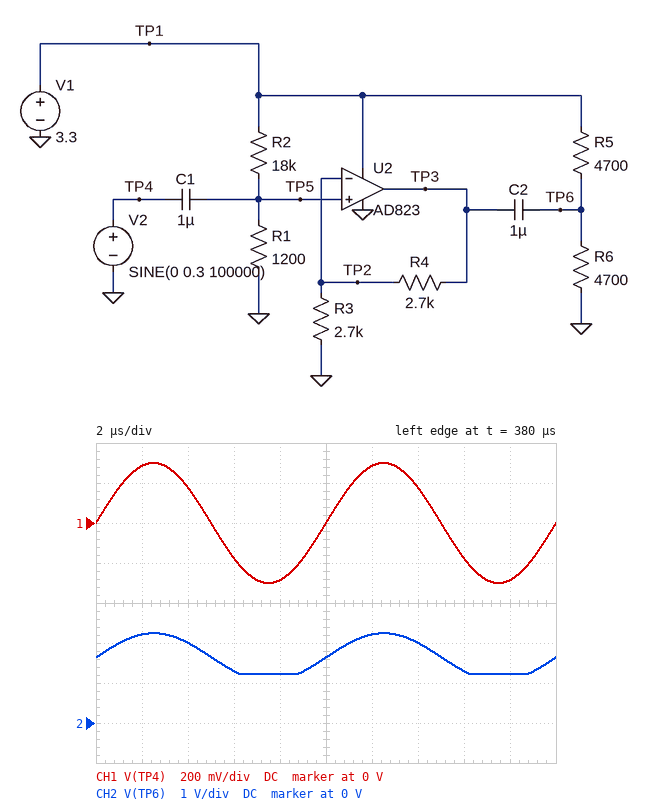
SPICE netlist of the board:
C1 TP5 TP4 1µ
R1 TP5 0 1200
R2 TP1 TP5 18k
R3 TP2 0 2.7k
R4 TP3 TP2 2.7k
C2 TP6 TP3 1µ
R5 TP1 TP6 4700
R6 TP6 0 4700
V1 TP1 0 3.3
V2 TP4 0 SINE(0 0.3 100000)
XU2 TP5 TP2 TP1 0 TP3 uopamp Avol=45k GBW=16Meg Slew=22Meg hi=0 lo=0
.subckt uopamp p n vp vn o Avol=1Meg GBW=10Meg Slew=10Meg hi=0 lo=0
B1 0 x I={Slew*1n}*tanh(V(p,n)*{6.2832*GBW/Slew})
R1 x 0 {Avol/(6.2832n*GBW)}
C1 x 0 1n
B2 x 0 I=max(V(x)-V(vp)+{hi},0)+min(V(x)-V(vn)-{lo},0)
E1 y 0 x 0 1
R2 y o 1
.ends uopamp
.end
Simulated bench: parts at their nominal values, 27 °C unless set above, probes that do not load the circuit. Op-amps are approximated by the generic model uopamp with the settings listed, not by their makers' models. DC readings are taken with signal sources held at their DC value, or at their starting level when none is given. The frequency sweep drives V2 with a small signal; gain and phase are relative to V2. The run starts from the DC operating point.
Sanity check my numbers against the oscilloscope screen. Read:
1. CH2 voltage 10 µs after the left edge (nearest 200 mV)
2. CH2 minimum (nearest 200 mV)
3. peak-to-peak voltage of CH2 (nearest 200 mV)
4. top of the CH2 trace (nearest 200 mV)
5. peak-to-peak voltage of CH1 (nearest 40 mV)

1.6 V
1.2 V
1.0 V
2.2 V
600 mV
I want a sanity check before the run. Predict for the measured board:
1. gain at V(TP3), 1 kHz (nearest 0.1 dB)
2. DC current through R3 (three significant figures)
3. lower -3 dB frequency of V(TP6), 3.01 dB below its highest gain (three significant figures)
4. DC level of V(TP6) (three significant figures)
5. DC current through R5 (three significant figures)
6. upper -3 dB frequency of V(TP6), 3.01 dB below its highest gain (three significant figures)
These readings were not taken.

5.9 dB
76.4 µA
167 Hz
1.65 V
351 µA
8.00 MHz
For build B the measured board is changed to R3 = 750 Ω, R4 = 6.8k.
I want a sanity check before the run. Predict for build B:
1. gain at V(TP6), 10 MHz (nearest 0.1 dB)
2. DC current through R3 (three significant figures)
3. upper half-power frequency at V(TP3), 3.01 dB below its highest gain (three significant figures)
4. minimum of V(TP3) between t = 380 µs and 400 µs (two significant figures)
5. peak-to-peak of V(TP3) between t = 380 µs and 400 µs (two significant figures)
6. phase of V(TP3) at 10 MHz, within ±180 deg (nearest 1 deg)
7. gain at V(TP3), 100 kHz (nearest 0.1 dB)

4.0 dB
275 µA
1.59 MHz
-8.0 mV
3.3 V
-81 deg
20.0 dB
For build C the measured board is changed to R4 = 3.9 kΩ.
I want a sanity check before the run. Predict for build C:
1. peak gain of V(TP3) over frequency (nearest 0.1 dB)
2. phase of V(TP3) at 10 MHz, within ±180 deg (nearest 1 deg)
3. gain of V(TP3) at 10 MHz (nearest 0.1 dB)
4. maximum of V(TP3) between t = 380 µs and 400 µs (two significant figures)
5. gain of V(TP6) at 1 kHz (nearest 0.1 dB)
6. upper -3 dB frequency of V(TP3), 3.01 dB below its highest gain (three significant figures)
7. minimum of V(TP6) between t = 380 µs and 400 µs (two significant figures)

7.8 dB
-57 deg
2.5 dB
1.2 V
7.7 dB
6.54 MHz
1.1 V
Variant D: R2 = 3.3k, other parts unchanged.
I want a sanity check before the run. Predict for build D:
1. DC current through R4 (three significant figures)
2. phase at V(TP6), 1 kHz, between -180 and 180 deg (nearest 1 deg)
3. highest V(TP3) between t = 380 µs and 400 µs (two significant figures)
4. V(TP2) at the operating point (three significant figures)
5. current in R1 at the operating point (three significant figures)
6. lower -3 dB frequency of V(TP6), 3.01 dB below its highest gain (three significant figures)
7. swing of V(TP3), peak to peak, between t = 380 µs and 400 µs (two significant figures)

326 µA
14 deg
2.4 V
880 mV
733 µA
202 Hz
1.2 V
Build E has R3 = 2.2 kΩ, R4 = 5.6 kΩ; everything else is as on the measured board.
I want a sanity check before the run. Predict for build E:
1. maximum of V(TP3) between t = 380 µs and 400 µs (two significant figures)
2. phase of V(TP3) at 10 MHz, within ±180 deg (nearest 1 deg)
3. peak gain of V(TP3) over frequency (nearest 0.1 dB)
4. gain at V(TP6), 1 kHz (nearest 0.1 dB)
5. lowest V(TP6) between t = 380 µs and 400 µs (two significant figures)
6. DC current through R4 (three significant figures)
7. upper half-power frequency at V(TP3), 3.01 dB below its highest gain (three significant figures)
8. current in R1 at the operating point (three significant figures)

1.8 V
-66 deg
11.0 dB
10.9 dB
900 mV
93.7 µA
4.51 MHz
172 µA
